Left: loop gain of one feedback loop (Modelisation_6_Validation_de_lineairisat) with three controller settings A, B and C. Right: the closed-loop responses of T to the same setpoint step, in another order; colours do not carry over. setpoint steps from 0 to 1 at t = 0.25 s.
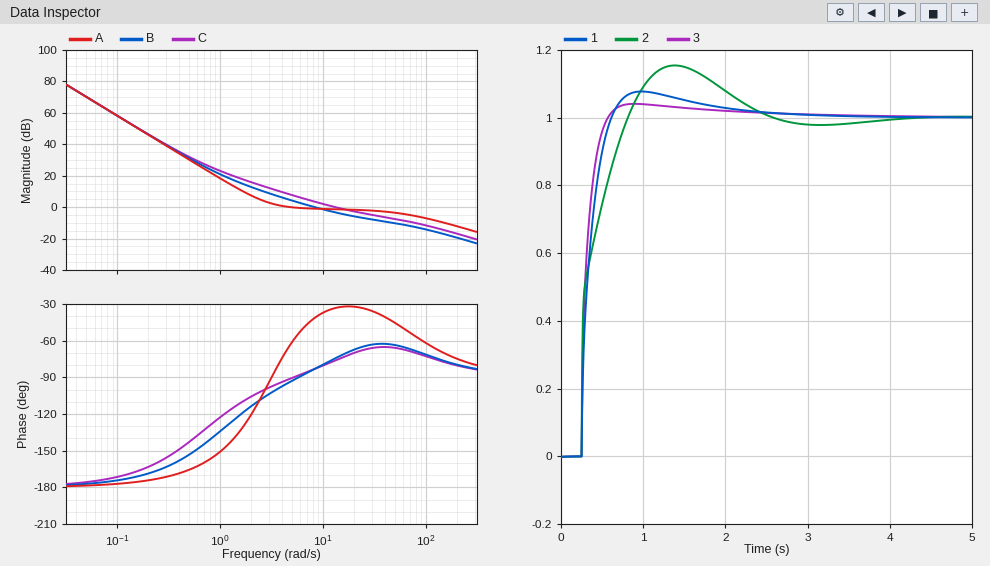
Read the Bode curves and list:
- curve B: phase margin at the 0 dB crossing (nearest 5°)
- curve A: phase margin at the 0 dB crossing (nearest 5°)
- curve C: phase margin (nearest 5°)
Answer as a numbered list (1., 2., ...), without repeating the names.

1. 95°
2. 115°
3. 105°
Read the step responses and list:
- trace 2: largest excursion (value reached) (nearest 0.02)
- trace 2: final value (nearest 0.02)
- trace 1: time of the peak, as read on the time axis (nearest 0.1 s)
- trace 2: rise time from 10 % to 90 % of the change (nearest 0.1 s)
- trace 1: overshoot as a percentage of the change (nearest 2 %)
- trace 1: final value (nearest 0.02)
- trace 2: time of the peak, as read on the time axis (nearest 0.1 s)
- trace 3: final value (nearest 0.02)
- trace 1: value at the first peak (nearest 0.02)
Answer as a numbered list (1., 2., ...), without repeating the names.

1. 1.16
2. 1.00
3. 1.0 s
4. 0.4 s
5. 8 %
6. 1.00
7. 1.4 s
8. 1.00
9. 1.08
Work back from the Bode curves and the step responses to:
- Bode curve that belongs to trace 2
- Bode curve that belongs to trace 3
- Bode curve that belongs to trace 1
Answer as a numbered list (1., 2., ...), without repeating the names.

1. A
2. C
3. B
